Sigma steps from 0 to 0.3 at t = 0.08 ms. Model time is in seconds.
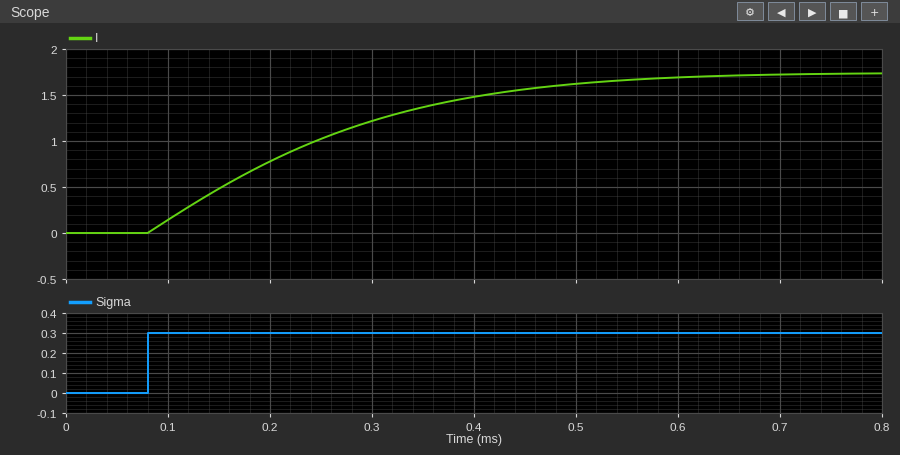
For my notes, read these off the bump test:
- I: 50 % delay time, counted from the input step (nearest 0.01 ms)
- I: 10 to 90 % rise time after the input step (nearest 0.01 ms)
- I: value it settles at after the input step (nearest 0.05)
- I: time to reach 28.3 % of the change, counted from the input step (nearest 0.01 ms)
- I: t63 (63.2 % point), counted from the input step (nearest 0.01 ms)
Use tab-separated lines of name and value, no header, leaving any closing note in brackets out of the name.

I: 50 % delay time, counted from the input step	0.14 ms
I: 10 to 90 % rise time after the input step	0.35 ms
I: value it settles at after the input step	1.75
I: time to reach 28.3 % of the change, counted from the input step	0.07 ms
I: t63 (63.2 % point), counted from the input step	0.19 ms
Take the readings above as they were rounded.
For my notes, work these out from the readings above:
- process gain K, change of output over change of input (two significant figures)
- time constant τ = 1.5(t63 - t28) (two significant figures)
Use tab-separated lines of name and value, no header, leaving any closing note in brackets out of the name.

process gain K, change of output over change of input	5.8
time constant τ = 1.5(t63 - t28)	0.18 ms
